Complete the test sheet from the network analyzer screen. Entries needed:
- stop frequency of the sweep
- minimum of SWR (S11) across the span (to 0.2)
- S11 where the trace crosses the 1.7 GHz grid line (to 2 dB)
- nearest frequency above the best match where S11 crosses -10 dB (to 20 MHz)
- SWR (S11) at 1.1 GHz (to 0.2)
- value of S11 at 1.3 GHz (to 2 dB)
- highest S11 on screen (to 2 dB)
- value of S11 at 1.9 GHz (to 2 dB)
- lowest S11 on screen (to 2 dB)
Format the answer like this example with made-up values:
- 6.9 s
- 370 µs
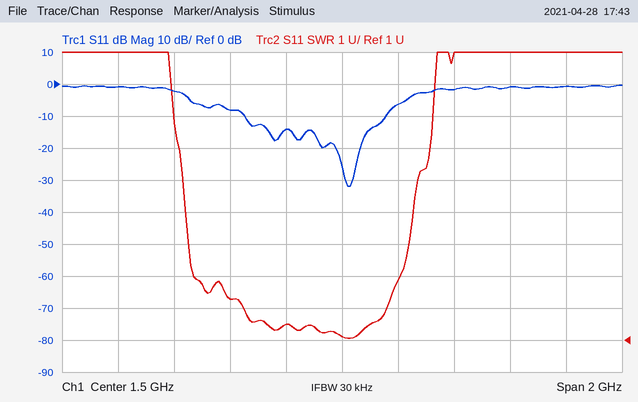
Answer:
- 2.5 GHz
- 1.0
- -6 dB
- 1.66 GHz
- 2.2
- -14 dB
- 0 dB
- -2 dB
- -32 dB
